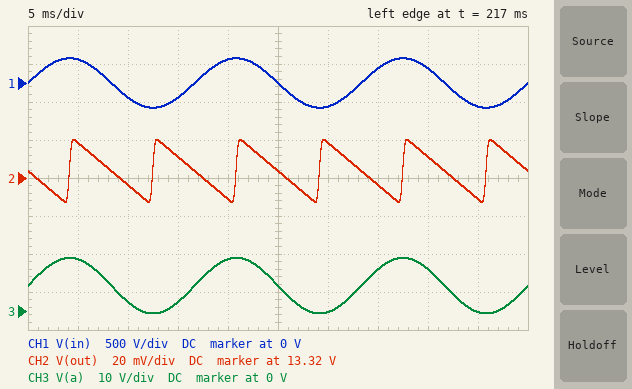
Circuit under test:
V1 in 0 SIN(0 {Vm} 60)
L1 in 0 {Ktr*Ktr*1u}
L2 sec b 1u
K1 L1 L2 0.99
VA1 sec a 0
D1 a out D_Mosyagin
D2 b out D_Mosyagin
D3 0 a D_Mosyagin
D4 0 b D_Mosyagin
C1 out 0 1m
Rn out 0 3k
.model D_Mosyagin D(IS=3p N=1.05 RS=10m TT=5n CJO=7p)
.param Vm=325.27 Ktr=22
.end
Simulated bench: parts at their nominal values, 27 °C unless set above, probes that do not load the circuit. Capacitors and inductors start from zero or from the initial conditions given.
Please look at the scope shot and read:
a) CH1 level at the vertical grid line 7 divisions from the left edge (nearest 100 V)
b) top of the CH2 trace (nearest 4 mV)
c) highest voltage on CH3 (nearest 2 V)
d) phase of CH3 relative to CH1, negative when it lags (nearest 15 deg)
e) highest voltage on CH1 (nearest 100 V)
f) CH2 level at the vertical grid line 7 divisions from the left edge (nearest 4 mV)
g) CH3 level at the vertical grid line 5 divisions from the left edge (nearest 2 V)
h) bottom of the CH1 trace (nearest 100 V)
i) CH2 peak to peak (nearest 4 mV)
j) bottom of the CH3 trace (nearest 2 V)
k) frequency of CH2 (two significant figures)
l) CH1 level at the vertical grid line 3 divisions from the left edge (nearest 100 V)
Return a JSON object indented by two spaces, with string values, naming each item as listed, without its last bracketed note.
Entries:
{
  "CH1 level at the vertical grid line 7 divisions from the left edge": "200 V",
  "top of the CH2 trace": "13.340 V",
  "highest voltage on CH3": "14 V",
  "phase of CH3 relative to CH1, negative when it lags": "0 deg",
  "highest voltage on CH1": "300 V",
  "CH2 level at the vertical grid line 7 divisions from the left edge": "13.316 V",
  "CH3 level at the vertical grid line 5 divisions from the left edge": "6 V",
  "bottom of the CH1 trace": "-300 V",
  "CH2 peak to peak": "32 mV",
  "bottom of the CH3 trace": "0 V",
  "frequency of CH2": "120 Hz",
  "CH1 level at the vertical grid line 3 divisions from the left edge": "-200 V"
}
